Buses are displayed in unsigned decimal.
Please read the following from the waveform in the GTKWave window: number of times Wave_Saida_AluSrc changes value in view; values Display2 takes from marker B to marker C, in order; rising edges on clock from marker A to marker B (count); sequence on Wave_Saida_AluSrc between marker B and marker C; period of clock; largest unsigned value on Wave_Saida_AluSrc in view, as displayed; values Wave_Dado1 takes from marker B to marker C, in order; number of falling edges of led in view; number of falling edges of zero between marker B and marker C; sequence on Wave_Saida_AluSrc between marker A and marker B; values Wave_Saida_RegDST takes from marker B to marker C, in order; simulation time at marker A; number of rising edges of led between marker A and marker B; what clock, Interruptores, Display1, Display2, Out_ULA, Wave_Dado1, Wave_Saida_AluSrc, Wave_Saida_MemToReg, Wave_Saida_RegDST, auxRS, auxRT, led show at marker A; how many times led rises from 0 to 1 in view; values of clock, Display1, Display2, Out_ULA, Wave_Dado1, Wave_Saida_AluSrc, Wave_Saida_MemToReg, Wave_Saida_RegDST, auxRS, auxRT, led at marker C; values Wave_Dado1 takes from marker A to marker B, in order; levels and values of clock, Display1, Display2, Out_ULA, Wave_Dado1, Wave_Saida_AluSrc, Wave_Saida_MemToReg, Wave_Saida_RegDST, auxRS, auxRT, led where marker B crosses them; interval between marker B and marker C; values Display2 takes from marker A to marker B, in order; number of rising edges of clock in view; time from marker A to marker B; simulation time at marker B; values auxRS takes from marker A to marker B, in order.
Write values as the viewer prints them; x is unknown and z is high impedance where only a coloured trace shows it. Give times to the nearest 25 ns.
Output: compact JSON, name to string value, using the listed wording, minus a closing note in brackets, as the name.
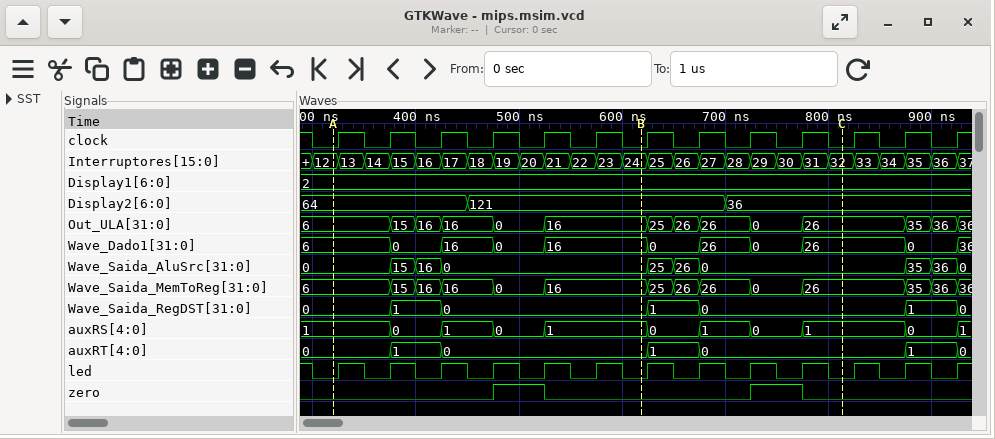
{"number of times Wave_Saida_AluSrc changes value in view": "9", "values Display2 takes from marker B to marker C, in order": "121, 36", "rising edges on clock from marker A to marker B": "6", "sequence on Wave_Saida_AluSrc between marker B and marker C": "0, 25, 26, 0", "period of clock": "50 ns", "largest unsigned value on Wave_Saida_AluSrc in view, as displayed": "36", "values Wave_Dado1 takes from marker B to marker C, in order": "16, 0, 26, 0, 26", "number of falling edges of led in view": "13", "number of falling edges of zero between marker B and marker C": "1", "sequence on Wave_Saida_AluSrc between marker A and marker B": "0, 15, 16, 0", "values Wave_Saida_RegDST takes from marker B to marker C, in order": "0, 1, 0", "simulation time at marker A": "325 ns", "number of rising edges of led between marker A and marker B": "6", "what clock, Interruptores, Display1, Display2, Out_ULA, Wave_Dado1, Wave_Saida_AluSrc, Wave_Saida_MemToReg, Wave_Saida_RegDST, auxRS, auxRT, led show at marker A": "clock=0, Interruptores=12, Display1=2, Display2=64, Out_ULA=6, Wave_Dado1=6, Wave_Saida_AluSrc=0, Wave_Saida_MemToReg=6, Wave_Saida_RegDST=0, auxRS=1, auxRT=0, led=0", "how many times led rises from 0 to 1 in view": "13", "values of clock, Display1, Display2, Out_ULA, Wave_Dado1, Wave_Saida_AluSrc, Wave_Saida_MemToReg, Wave_Saida_RegDST, auxRS, auxRT, led at marker C": "clock=0, Display1=2, Display2=36, Out_ULA=26, Wave_Dado1=26, Wave_Saida_AluSrc=0, Wave_Saida_MemToReg=26, Wave_Saida_RegDST=0, auxRS=1, auxRT=0, led=0", "values Wave_Dado1 takes from marker A to marker B, in order": "6, 0, 16, 0, 16", "levels and values of clock, Display1, Display2, Out_ULA, Wave_Dado1, Wave_Saida_AluSrc, Wave_Saida_MemToReg, Wave_Saida_RegDST, auxRS, auxRT, led where marker B crosses them": "clock=0, Display1=2, Display2=121, Out_ULA=16, Wave_Dado1=16, Wave_Saida_AluSrc=0, Wave_Saida_MemToReg=16, Wave_Saida_RegDST=0, auxRS=1, auxRT=0, led=0", "interval between marker B and marker C": "200 ns", "values Display2 takes from marker A to marker B, in order": "64, 121", "number of rising edges of clock in view": "13", "time from marker A to marker B": "300 ns", "simulation time at marker B": "625 ns", "values auxRS takes from marker A to marker B, in order": "1, 0, 1, 0, 1"}
